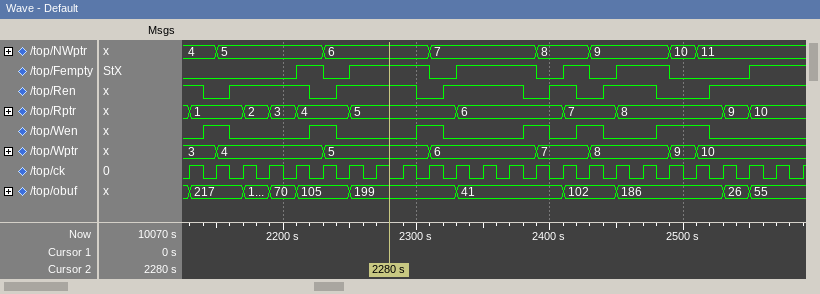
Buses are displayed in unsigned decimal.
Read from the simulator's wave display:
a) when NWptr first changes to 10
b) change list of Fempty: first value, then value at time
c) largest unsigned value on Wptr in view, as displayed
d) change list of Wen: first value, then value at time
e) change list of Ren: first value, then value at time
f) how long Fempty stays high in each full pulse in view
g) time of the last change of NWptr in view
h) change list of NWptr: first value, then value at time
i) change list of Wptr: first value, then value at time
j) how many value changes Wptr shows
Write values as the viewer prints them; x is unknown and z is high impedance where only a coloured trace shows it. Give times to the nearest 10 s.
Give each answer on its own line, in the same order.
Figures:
2490 s
0, 1 at 2210 s, 0 at 2230 s, 1 at 2250 s, 0 at 2310 s, 1 at 2330 s, 0 at 2390 s, 1 at 2410 s, 0 at 2430 s, 1 at 2450 s, 0 at 2490 s, 1 at 2550 s
10
0, 1 at 2140 s, 0 at 2160 s, 1 at 2220 s, 0 at 2240 s, 1 at 2300 s, 0 at 2320 s, 1 at 2380 s, 0 at 2400 s, 1 at 2420 s, 0 at 2440 s, 1 at 2480 s, 0 at 2520 s
1, 0 at 2140 s, 1 at 2160 s, 0 at 2220 s, 1 at 2240 s, 0 at 2300 s, 1 at 2320 s, 0 at 2380 s, 1 at 2400 s, 0 at 2420 s, 1 at 2440 s, 0 at 2480 s, 1 at 2520 s
20 s, 60 s, 60 s, 20 s, 40 s
2510 s
4, 5 at 2150 s, 6 at 2230 s, 7 at 2310 s, 8 at 2390 s, 9 at 2430 s, 10 at 2490 s, 11 at 2510 s
3, 4 at 2150 s, 5 at 2230 s, 6 at 2310 s, 7 at 2390 s, 8 at 2430 s, 9 at 2490 s, 10 at 2510 s
7
